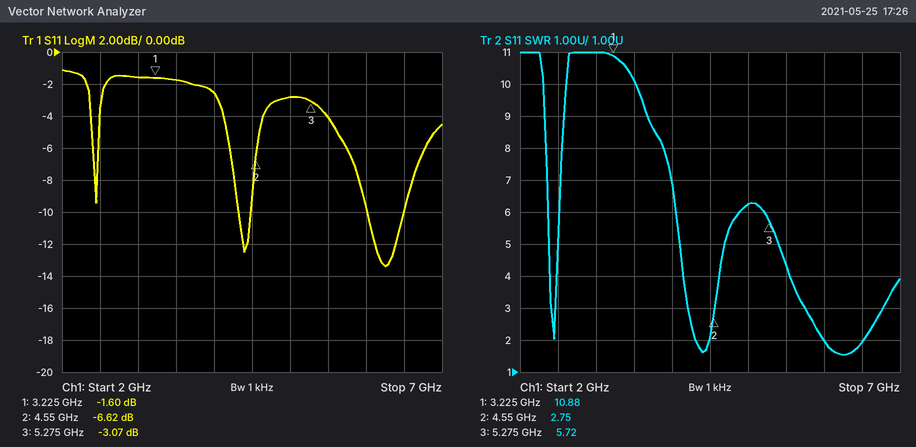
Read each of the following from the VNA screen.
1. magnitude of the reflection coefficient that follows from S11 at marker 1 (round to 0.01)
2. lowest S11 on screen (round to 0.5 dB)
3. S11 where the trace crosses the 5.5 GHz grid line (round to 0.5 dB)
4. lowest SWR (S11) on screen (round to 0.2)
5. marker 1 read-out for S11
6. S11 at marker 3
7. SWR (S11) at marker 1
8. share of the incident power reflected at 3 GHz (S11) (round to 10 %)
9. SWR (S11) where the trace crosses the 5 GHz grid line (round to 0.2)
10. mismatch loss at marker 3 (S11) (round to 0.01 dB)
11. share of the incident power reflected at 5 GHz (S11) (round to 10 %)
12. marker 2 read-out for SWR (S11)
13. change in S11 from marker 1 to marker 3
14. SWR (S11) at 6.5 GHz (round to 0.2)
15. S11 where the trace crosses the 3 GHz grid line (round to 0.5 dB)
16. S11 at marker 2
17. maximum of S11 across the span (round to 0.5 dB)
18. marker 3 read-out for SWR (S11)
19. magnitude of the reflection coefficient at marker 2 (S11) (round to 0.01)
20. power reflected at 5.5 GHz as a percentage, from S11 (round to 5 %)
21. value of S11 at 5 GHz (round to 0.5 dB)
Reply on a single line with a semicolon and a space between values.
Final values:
0.83; -13.5 dB; -4.0 dB; 1.6; -1.60 dB; -3.07 dB; 10.88; 70 %; 6.2; 2.95 dB; 50 %; 2.75; -1.47 dB; 2.0; -1.5 dB; -6.62 dB; -1.0 dB; 5.72; 0.47; 40 %; -3.0 dB
